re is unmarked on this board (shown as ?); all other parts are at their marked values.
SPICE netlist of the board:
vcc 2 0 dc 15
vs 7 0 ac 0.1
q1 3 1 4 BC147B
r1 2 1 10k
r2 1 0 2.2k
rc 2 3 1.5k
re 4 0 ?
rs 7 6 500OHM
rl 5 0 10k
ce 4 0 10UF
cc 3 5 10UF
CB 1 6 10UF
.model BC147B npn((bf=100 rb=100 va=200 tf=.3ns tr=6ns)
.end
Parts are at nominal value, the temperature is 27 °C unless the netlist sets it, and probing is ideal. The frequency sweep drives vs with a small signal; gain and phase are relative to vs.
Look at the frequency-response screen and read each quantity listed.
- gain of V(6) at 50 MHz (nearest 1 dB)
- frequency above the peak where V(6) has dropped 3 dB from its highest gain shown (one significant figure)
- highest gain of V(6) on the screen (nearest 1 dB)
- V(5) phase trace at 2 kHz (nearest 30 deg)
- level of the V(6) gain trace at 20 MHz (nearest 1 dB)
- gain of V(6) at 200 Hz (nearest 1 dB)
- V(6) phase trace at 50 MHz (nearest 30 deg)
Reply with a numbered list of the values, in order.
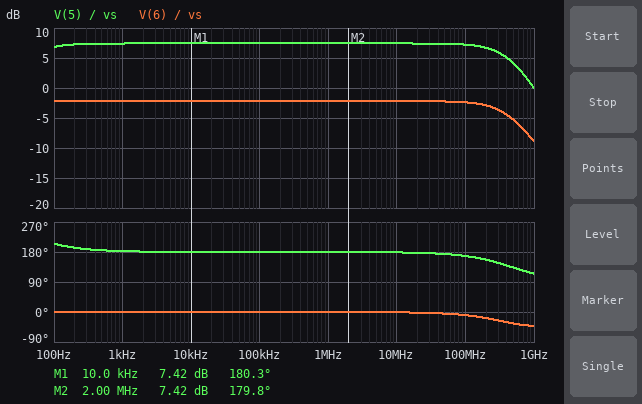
1. -2 dB
2. 500 MHz
3. -2 dB
4. 180 deg
5. -2 dB
6. -2 dB
7. 0 deg
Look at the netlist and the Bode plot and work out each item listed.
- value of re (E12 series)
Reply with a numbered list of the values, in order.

1. 33 kΩ
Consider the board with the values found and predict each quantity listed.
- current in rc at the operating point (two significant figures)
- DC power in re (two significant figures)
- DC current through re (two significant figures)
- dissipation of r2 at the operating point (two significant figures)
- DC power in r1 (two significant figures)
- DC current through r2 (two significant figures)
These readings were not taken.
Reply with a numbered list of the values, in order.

1. 60 µA
2. 120 µW
3. 61 µA
4. 3.3 mW
5. 15 mW
6. 1.2 mA
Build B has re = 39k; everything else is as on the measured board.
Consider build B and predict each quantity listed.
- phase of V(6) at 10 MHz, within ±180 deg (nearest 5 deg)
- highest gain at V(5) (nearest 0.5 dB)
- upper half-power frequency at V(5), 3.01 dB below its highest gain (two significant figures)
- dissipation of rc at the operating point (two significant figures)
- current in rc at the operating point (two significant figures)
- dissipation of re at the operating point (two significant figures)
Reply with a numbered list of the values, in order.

1. 0 deg
2. 6.0 dB
3. 550 MHz
4. 3.9 µW
5. 51 µA
6. 100 µW
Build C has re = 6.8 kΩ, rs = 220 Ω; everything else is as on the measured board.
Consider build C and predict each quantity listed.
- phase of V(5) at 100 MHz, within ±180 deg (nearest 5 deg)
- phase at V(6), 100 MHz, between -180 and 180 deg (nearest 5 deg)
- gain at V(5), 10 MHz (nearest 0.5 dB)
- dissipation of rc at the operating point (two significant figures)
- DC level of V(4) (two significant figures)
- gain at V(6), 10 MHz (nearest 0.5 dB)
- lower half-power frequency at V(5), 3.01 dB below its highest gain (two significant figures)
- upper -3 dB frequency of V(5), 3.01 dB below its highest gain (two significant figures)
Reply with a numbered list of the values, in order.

1. 150 deg
2. -20 deg
3. 22.0 dB
4. 120 µW
5. 2.0 V
6. -1.0 dB
7. 180 Hz
8. 170 MHz
